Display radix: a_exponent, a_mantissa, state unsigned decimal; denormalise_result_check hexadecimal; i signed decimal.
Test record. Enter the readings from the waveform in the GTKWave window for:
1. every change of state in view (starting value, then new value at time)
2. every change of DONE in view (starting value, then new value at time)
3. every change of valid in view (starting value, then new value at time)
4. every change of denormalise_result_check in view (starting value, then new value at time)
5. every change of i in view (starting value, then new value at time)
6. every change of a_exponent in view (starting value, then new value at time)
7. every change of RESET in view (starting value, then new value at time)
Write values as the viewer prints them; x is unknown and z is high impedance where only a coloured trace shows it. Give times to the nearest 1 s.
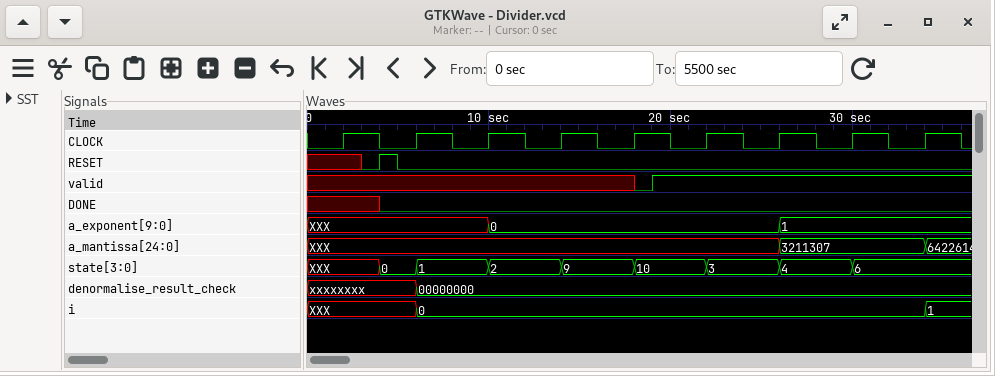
XXX, 0 at 4 s, 1 at 6 s, 2 at 10 s, 9 at 14 s, 10 at 18 s, 3 at 22 s, 4 at 26 s, 6 at 30 s
x, 0 at 4 s
x, 0 at 18 s, 1 at 19 s
xxxxxxxx, 00000000 at 6 s
XXX, 0 at 6 s, 1 at 34 s
XXX, 0 at 10 s, 1 at 26 s
x, 0 at 3 s, 1 at 4 s, 0 at 5 s
